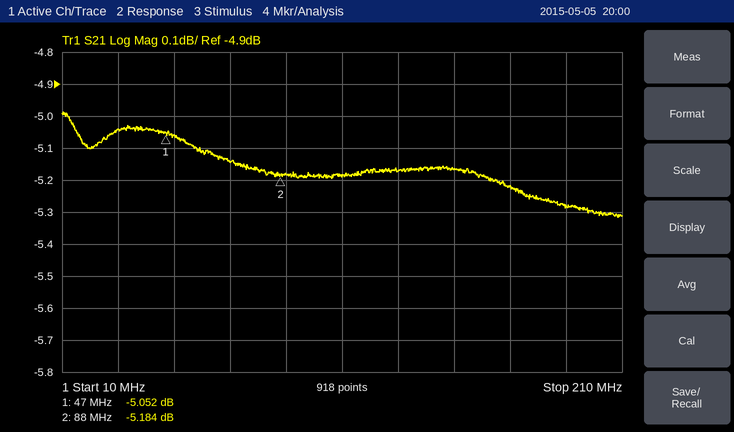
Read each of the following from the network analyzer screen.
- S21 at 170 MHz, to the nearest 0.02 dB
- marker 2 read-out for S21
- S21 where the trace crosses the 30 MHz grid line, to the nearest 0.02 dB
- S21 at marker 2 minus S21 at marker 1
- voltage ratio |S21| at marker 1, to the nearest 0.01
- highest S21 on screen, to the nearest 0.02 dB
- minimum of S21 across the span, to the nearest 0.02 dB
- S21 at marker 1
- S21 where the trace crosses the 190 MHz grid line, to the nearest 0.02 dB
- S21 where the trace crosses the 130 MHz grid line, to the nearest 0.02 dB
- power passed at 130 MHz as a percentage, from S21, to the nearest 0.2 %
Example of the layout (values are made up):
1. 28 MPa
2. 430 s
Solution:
1. -5.22 dB
2. -5.184 dB
3. -5.04 dB
4. -0.132 dB
5. 0.56
6. -4.98 dB
7. -5.32 dB
8. -5.052 dB
9. -5.28 dB
10. -5.18 dB
11. 30.4 %
